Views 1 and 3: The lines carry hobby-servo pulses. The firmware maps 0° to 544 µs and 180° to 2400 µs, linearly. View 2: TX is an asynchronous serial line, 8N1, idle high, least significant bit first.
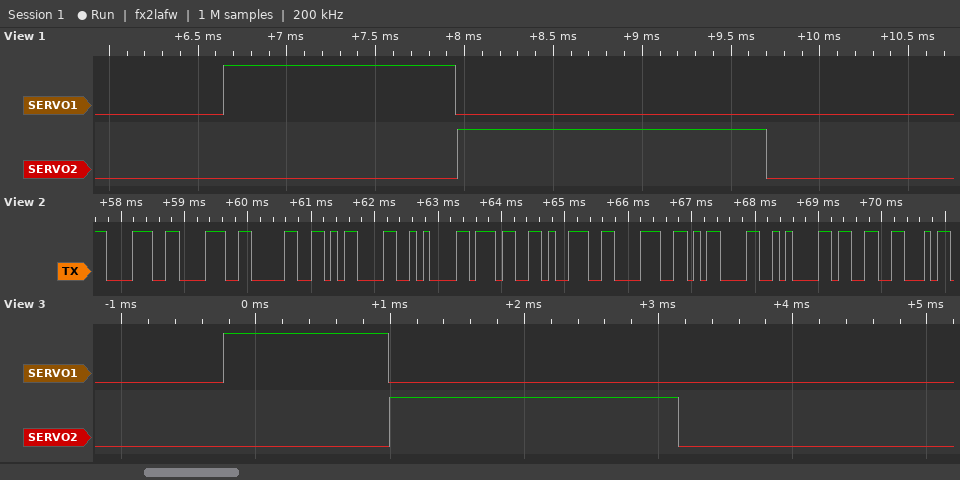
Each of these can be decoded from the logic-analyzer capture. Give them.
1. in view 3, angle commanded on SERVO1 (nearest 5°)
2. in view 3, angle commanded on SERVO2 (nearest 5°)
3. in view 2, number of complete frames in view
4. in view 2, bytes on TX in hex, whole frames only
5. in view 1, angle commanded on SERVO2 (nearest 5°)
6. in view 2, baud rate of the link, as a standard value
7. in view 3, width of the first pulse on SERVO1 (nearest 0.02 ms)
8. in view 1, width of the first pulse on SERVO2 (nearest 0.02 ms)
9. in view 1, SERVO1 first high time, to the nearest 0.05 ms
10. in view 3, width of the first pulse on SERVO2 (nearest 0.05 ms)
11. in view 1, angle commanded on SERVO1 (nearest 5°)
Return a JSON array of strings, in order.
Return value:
["65°", "155°", "11", "38 38 30 0D 0A 37 39 38 0D 0A 33", "115°", "9600 baud", "1.22 ms", "1.74 ms", "1.30 ms", "2.15 ms", "75°"]
